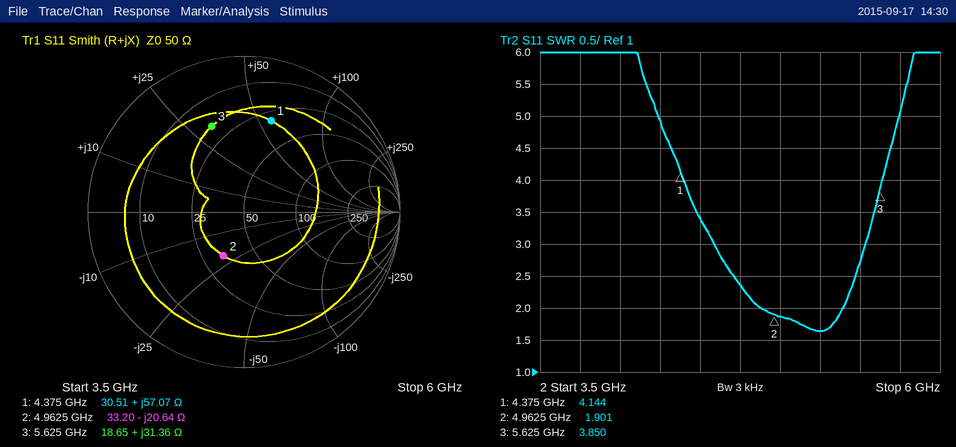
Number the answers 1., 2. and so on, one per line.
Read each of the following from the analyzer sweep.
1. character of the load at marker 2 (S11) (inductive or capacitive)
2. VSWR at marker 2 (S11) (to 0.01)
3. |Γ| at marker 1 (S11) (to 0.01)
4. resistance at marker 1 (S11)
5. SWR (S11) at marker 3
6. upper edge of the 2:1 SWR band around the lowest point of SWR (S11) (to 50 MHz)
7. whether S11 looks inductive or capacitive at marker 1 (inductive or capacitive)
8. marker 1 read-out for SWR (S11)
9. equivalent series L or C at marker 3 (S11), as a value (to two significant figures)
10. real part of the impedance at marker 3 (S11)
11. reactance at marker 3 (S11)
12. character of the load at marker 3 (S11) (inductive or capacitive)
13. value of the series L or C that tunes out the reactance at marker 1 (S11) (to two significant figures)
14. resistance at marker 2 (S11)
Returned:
1. capacitive
2. 1.90
3. 0.61
4. 30.51 Ω
5. 3.850
6. 5.40 GHz
7. inductive
8. 4.144
9. 890 pH
10. 18.65 Ω
11. +31.36 Ω
12. inductive
13. 640 fF
14. 33.20 Ω
